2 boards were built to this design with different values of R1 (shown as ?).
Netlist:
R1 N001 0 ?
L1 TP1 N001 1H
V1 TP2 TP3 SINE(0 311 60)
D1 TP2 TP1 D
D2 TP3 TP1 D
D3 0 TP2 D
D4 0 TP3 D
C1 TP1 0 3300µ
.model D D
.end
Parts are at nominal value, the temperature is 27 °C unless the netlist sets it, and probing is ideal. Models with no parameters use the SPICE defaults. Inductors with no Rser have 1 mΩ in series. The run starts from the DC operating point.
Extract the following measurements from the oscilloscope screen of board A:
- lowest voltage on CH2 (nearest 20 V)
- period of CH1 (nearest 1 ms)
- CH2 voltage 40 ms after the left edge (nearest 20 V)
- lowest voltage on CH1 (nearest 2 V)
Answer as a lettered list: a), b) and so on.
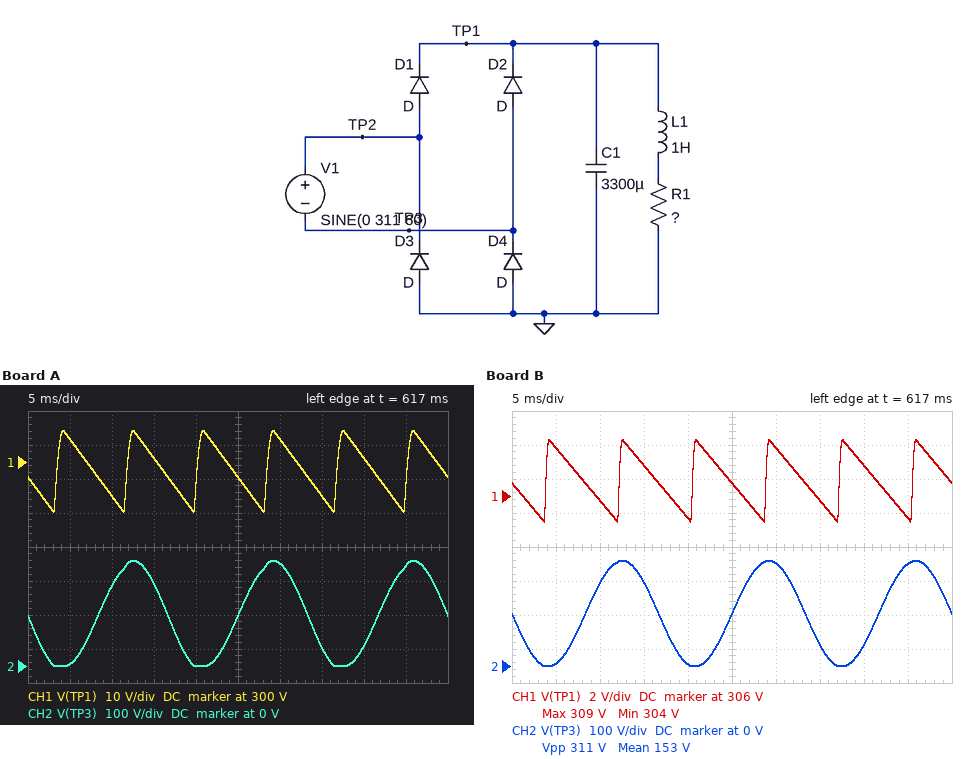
a) 0 V
b) 8 ms
c) 60 V
d) 286 V
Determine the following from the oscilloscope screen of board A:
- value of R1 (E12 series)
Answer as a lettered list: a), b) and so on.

a) 27 Ω
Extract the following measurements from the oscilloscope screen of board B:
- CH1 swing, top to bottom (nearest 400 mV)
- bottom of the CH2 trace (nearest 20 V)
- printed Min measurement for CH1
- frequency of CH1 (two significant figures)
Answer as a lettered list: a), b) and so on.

a) 4.8 V
b) 0 V
c) 304 V
d) 120 Hz
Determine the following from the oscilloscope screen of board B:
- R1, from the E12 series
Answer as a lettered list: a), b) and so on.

a) 150 Ω
